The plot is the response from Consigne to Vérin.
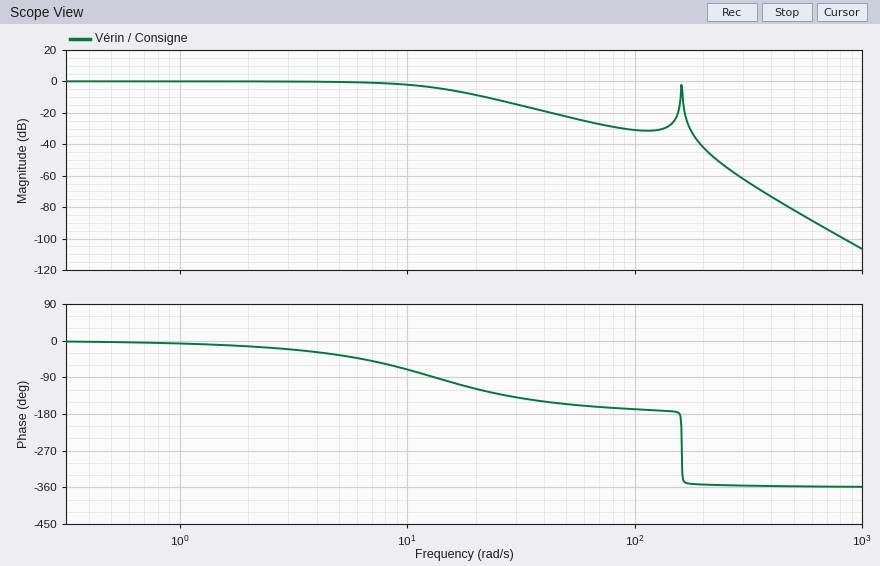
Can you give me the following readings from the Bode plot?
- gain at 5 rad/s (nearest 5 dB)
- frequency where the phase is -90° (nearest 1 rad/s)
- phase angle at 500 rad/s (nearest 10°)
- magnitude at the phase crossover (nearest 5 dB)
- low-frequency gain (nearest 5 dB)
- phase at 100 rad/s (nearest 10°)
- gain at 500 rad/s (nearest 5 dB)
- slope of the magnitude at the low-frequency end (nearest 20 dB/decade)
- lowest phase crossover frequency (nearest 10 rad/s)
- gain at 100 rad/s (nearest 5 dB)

0 dB
13 rad/s
-360°
-15 dB
0 dB
-170°
-80 dB
0 dB/decade
160 rad/s
-30 dB
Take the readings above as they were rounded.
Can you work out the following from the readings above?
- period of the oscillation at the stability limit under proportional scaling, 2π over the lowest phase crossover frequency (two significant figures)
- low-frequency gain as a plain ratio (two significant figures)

0.039 s
1.0
